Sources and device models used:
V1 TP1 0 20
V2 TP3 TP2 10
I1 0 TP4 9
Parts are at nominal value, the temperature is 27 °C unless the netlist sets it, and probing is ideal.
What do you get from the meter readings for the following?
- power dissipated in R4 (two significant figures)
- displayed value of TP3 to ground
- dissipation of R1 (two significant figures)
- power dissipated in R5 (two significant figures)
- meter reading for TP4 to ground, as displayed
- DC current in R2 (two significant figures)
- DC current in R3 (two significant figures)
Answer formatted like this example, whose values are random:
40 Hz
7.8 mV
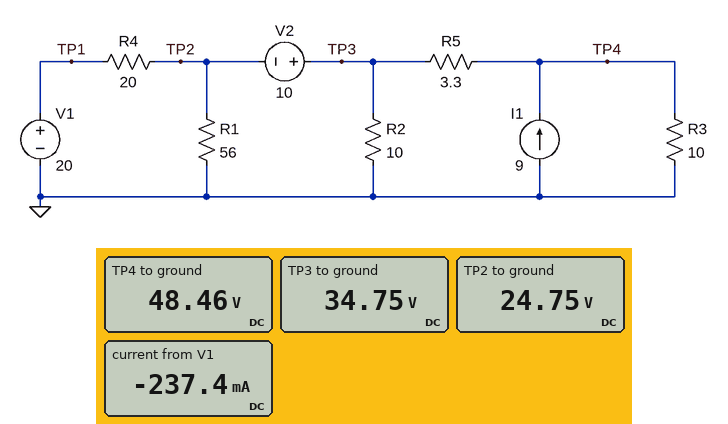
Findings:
1.1 W
34.75 V
11 W
57 W
48.46 V
3.5 A
4.8 A
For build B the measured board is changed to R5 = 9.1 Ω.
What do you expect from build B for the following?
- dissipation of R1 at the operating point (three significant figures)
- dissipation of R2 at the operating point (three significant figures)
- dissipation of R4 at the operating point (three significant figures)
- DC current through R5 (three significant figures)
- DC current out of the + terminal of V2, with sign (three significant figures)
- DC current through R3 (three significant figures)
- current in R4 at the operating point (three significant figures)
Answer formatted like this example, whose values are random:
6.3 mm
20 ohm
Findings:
6.46 W
84.2 W
48.0 mW
3.19 A
-291 mA
5.81 A
49.0 mA
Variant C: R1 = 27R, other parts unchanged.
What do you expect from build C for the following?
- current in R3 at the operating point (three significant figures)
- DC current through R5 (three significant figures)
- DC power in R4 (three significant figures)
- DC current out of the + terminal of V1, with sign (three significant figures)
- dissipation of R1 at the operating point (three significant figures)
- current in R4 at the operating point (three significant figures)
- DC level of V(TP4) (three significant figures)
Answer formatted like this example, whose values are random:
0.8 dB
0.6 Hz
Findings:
4.71 A
4.29 A
432 mW
-147 mA
19.5 W
147 mA
47.1 V
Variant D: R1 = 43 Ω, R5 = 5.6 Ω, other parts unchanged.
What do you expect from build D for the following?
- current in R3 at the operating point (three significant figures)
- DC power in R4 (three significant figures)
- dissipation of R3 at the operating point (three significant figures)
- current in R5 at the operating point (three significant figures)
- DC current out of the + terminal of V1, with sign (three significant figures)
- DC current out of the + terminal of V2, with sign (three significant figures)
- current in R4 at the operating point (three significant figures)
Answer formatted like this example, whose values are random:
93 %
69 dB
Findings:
5.26 A
129 mW
276 W
3.74 A
-80.3 mA
-583 mA
80.3 mA
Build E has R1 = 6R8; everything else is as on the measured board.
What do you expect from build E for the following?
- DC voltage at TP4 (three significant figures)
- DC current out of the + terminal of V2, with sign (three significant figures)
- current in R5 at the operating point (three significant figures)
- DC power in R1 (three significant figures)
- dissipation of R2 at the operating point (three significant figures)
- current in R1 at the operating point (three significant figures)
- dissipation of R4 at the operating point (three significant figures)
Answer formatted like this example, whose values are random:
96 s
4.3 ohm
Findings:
42.0 V
-2.18 A
4.80 A
38.4 W
68.4 W
2.38 A
738 mW
